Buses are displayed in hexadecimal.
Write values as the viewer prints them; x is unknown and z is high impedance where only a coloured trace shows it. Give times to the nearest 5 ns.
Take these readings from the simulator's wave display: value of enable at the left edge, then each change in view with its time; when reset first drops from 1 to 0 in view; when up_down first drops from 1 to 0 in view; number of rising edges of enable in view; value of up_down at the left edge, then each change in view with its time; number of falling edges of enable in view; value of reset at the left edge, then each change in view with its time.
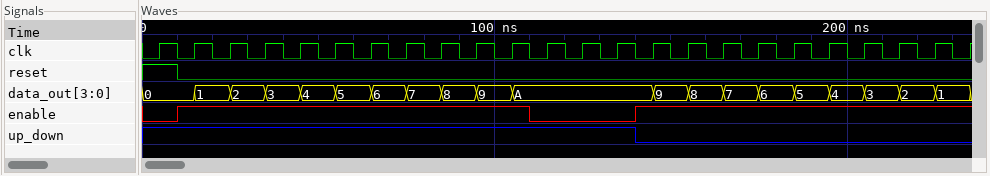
0, 1 at 10 ns, 0 at 110 ns, 1 at 140 ns
10 ns
140 ns
2
1, 0 at 140 ns
1
1, 0 at 10 ns
